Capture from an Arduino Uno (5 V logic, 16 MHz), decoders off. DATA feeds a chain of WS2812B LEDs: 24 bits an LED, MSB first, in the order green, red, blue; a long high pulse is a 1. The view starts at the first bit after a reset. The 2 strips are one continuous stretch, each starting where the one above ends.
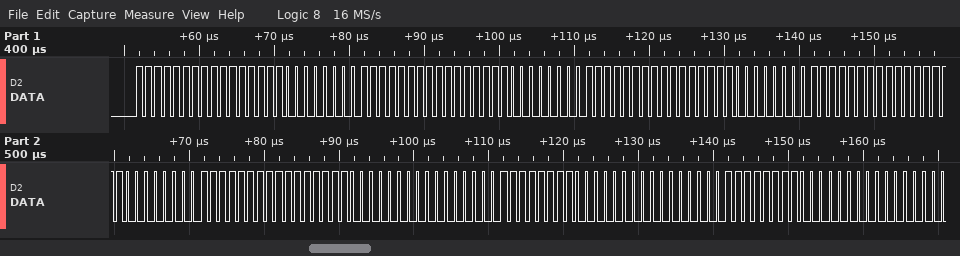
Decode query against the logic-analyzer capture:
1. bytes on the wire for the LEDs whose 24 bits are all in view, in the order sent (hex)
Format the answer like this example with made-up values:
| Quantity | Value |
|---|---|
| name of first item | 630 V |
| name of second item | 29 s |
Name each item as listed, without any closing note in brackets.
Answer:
| Quantity | Value |
|---|---|
| bytes on the wire for the LEDs whose 24 bits are all in view, in the order sent | FF FF 00 FF FF 00 FF FF 00 FF FF 00 FF FF 00 00 FF 00 00 FF 00 |
